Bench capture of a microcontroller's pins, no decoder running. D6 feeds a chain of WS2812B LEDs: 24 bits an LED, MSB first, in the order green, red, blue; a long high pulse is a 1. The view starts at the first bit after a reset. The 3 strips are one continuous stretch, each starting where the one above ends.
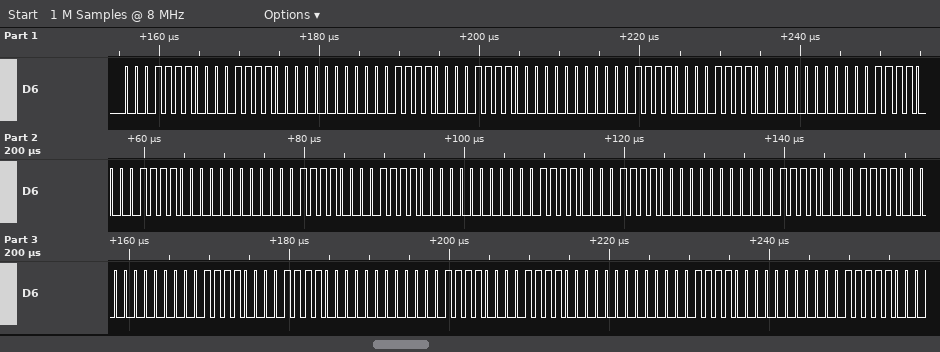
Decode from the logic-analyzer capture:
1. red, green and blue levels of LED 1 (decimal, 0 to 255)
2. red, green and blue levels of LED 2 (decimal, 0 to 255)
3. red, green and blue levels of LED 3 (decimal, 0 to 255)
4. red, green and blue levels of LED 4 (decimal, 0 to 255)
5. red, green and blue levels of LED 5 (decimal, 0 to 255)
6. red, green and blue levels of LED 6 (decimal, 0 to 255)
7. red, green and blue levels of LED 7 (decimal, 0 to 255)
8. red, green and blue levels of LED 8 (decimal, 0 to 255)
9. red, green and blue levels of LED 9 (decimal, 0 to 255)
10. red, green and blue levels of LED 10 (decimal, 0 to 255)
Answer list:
30, 30, 0
30, 30, 0
30, 30, 0
30, 30, 0
30, 30, 0
30, 30, 0
30, 30, 0
30, 30, 0
30, 30, 0
0, 15, 31
